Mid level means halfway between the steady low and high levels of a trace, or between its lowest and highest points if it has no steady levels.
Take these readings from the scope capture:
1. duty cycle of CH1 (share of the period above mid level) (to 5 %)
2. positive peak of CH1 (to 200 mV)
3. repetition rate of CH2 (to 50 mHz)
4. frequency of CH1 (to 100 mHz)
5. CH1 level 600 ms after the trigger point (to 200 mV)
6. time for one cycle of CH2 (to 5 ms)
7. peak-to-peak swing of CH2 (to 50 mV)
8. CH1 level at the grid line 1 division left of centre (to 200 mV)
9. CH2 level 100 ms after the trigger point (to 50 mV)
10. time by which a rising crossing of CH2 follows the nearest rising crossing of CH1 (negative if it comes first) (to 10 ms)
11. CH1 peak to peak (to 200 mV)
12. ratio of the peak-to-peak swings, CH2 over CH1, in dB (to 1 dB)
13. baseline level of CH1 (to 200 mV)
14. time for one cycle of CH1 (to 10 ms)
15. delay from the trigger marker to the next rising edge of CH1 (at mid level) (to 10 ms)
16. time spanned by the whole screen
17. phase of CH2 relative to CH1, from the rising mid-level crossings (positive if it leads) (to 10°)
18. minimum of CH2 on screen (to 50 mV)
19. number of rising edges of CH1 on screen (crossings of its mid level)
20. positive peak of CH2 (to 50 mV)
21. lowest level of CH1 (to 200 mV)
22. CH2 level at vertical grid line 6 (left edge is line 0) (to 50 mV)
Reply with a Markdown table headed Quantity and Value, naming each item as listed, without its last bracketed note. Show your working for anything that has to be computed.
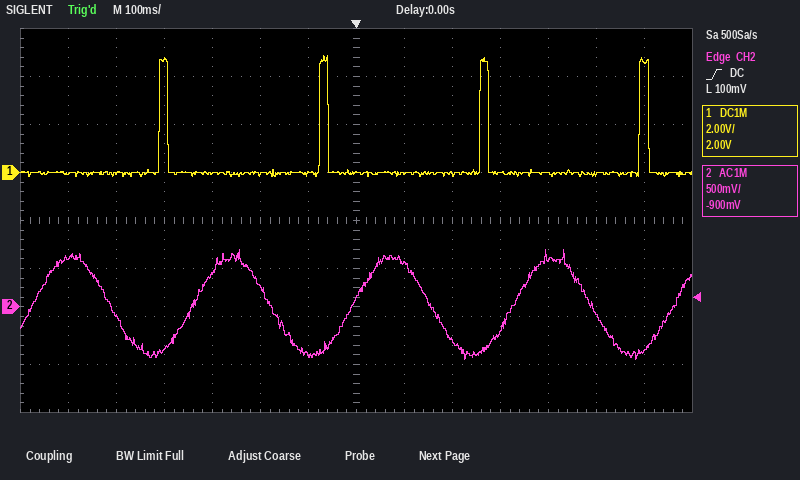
| Quantity | Value |
|---|---|
| duty cycle of CH1 (share of the period above mid level) | 5 % |
| positive peak of CH1 | 4.8 V |
| repetition rate of CH2 | 1 / 335 ms ≈ 2.99 Hz, so 3.00 Hz to the nearest 50 mHz |
| frequency of CH1 | 1 / 330 ms ≈ 3.0 Hz |
| CH1 level 600 ms after the trigger point | 4.6 V |
| time for one cycle of CH2 | 335 ms |
| peak-to-peak swing of CH2 | 600 mV − (-550 mV) = 1.15 V |
| CH1 level at the grid line 1 division left of centre | 0.0 V |
| CH2 level 100 ms after the trigger point | 450 mV |
| time by which a rising crossing of CH2 follows the nearest rising crossing of CH1 (negative if it comes first) | +70 ms |
| CH1 peak to peak | 4.8 V − (-200 mV) = 5.0 V |
| ratio of the peak-to-peak swings, CH2 over CH1, in dB | 20 log10(1.15 V / 5.0 V) ≈ -13 dB |
| baseline level of CH1 | 0.0 V |
| time for one cycle of CH1 | 330 ms |
| delay from the trigger marker to the next rising edge of CH1 (at mid level) | 260 ms |
| time spanned by the whole screen | 1.4 s |
| phase of CH2 relative to CH1, from the rising mid-level crossings (positive if it leads) | −360° × (+70 ms) / 330 ms ≈ -76.4°, so -80° to the nearest 10° |
| minimum of CH2 on screen | -550 mV |
| number of rising edges of CH1 on screen | 4 |
| positive peak of CH2 | 600 mV |
| lowest level of CH1 | -200 mV |
| CH2 level at vertical grid line 6 (left edge is line 0) | -500 mV |
